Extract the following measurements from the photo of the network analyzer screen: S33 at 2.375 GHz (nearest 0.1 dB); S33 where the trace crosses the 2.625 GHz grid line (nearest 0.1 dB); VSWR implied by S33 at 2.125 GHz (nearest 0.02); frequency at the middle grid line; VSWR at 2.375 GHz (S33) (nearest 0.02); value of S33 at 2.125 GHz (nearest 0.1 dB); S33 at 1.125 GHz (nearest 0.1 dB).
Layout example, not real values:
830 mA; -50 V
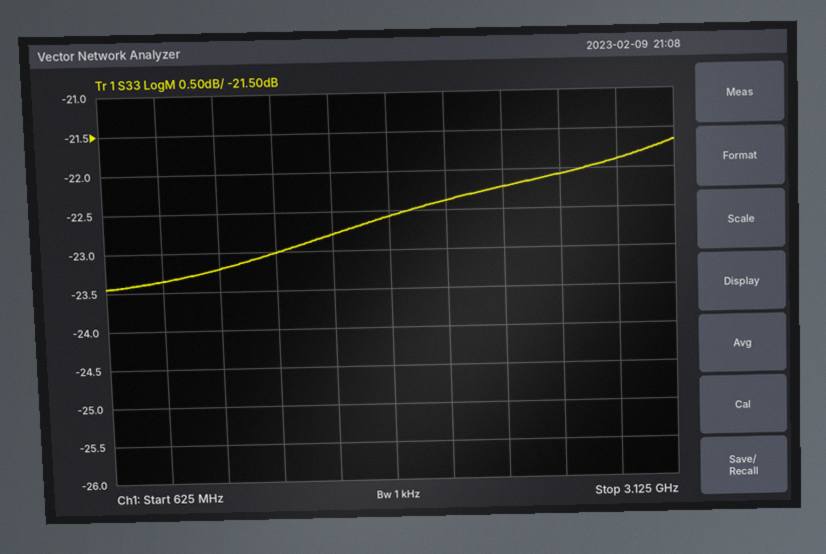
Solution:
-22.2 dB; -22.1 dB; 1.16; 1.875 GHz; 1.16; -22.4 dB; -23.2 dB
